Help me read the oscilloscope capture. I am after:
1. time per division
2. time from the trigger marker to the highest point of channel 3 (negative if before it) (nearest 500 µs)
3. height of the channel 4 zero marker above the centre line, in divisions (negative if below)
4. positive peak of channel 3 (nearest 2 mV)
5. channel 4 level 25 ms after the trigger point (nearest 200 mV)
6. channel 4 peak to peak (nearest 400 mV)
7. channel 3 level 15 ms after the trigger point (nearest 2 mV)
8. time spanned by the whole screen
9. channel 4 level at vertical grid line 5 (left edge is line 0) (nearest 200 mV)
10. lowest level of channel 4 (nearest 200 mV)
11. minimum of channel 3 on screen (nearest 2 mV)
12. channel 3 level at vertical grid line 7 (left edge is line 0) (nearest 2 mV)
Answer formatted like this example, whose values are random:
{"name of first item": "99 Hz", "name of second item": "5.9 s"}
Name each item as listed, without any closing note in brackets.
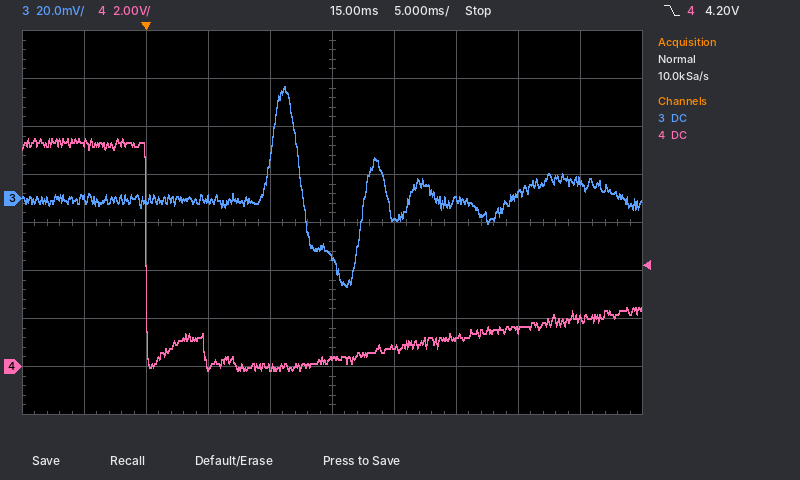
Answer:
{"time per division": "5 ms", "time from the trigger marker to the highest point of channel 3 (negative if before it)": "+11.0 ms", "height of the channel 4 zero marker above the centre line, in divisions": "-3.0 div", "positive peak of channel 3": "46 mV", "channel 4 level 25 ms after the trigger point": "1.2 V", "channel 4 peak to peak": "9.6 V", "channel 3 level 15 ms after the trigger point": "-24 mV", "time spanned by the whole screen": "50 ms", "channel 4 level at vertical grid line 5 (left edge is line 0)": "400 mV", "lowest level of channel 4": "-200 mV", "minimum of channel 3 on screen": "-36 mV", "channel 3 level at vertical grid line 7 (left edge is line 0)": "0 mV"}
